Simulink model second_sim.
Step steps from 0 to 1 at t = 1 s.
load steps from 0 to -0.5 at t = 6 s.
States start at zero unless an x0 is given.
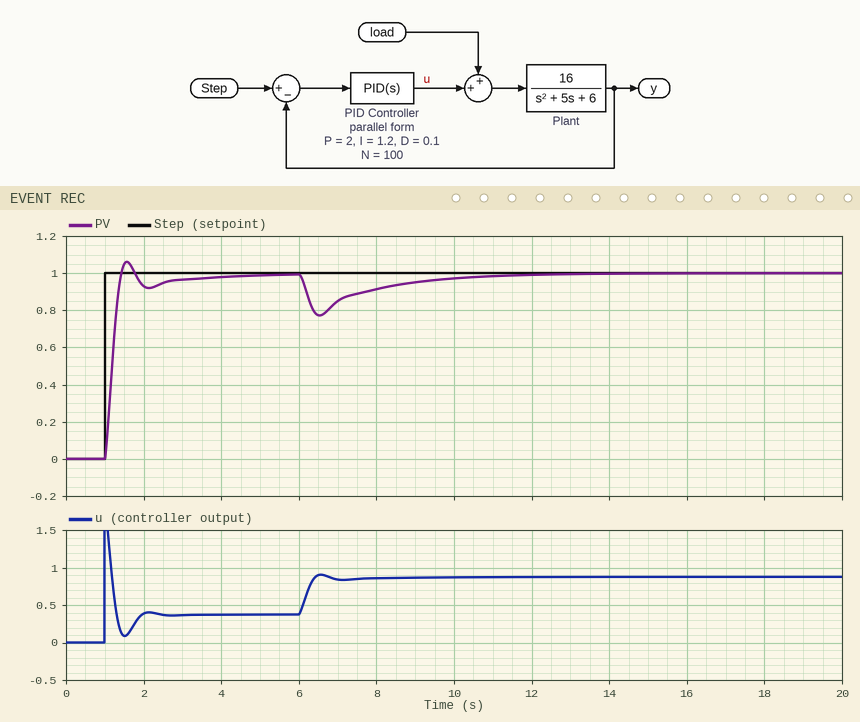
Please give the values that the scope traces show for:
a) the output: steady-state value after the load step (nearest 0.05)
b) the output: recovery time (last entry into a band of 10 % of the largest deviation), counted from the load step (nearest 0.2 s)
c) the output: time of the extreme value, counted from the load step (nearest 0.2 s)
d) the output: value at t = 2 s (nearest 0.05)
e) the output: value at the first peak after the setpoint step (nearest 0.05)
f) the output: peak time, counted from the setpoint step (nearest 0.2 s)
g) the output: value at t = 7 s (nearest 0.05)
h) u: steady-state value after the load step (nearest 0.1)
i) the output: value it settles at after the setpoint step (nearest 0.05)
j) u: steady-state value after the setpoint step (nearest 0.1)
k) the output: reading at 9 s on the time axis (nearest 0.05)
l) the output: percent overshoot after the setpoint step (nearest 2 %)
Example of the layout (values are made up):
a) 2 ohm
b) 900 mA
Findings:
a) 1.00
b) 4.4 s
c) 0.6 s
d) 0.95
e) 1.05
f) 0.6 s
g) 0.85
h) 0.9
i) 1.00
j) 0.4
k) 0.95
l) 6 %
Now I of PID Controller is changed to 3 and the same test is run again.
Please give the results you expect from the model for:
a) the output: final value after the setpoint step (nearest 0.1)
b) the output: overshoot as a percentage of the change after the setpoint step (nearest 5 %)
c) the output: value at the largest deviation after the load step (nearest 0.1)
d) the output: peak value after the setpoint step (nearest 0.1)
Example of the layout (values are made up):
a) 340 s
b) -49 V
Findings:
a) 1.0
b) 20 %
c) 0.8
d) 1.2
